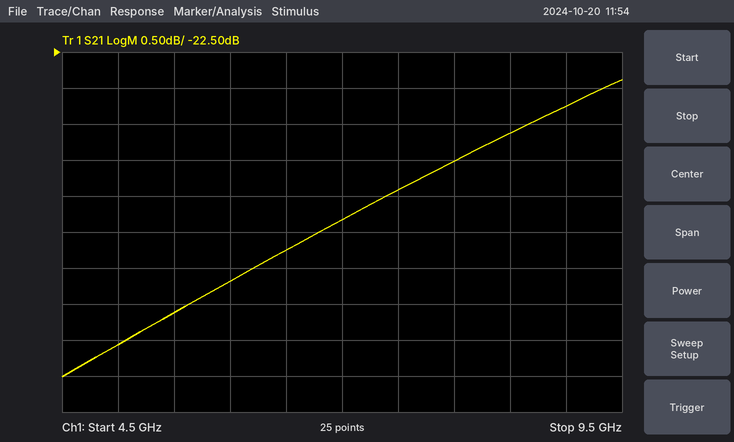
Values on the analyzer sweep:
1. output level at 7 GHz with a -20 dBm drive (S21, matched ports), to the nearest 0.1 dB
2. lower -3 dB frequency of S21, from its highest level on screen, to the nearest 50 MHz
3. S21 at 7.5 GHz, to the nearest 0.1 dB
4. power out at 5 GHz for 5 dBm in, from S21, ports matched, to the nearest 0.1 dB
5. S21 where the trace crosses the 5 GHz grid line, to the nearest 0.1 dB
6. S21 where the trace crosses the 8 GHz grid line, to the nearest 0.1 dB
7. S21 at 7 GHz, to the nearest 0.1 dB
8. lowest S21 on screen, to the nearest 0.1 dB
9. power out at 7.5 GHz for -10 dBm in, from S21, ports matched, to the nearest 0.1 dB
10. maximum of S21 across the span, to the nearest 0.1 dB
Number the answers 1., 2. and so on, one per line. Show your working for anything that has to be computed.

1. -20 dBm + (-24.8 dB) = -44.8 dBm
2. 5.75 GHz
3. -24.4 dB
4. 5 dBm + (-26.6 dB) = -21.6 dBm
5. -26.6 dB
6. -24.0 dB
7. -24.8 dB
8. -27.0 dB
9. -10 dBm + (-24.4 dB) = -34.4 dBm
10. -22.9 dB
